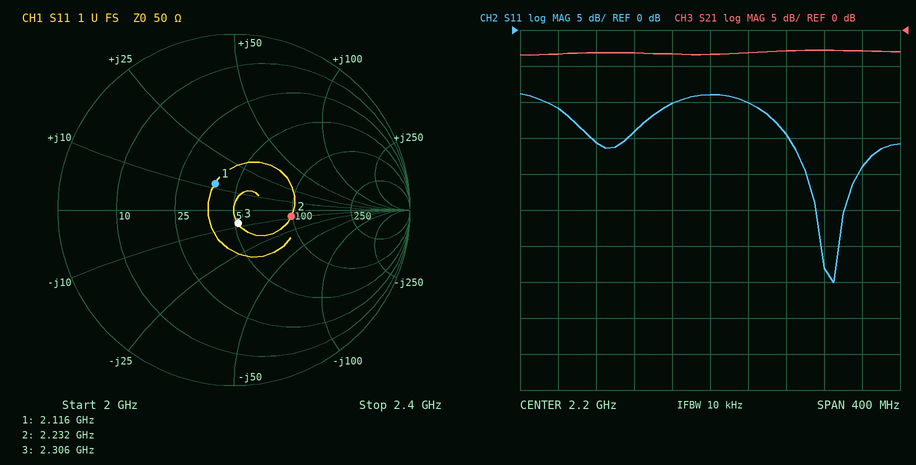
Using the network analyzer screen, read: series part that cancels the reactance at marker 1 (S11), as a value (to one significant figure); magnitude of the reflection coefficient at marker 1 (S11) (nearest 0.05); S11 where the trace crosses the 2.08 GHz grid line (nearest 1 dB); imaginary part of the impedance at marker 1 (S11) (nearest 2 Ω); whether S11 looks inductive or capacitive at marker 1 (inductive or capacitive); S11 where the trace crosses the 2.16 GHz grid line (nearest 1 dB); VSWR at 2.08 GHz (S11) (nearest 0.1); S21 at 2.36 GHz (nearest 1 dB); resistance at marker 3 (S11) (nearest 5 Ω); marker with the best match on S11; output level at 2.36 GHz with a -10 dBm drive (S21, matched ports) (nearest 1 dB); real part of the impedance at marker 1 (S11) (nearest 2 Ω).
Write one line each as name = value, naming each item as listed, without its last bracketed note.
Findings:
series part that cancels the reactance at marker 1 (S11), as a value = 6 pF
magnitude of the reflection coefficient at marker 1 (S11) = 0.20
S11 where the trace crosses the 2.08 GHz grid line = -16 dB
imaginary part of the impedance at marker 1 (S11) = +12 Ω
whether S11 looks inductive or capacitive at marker 1 = inductive
S11 where the trace crosses the 2.16 GHz grid line = -10 dB
VSWR at 2.08 GHz (S11) = 1.4
S21 at 2.36 GHz = -3 dB
resistance at marker 3 (S11) = 50 Ω
marker with the best match on S11 = marker 3
output level at 2.36 GHz with a -10 dBm drive (S21, matched ports) = -13 dBm
real part of the impedance at marker 1 (S11) = 38 Ω
